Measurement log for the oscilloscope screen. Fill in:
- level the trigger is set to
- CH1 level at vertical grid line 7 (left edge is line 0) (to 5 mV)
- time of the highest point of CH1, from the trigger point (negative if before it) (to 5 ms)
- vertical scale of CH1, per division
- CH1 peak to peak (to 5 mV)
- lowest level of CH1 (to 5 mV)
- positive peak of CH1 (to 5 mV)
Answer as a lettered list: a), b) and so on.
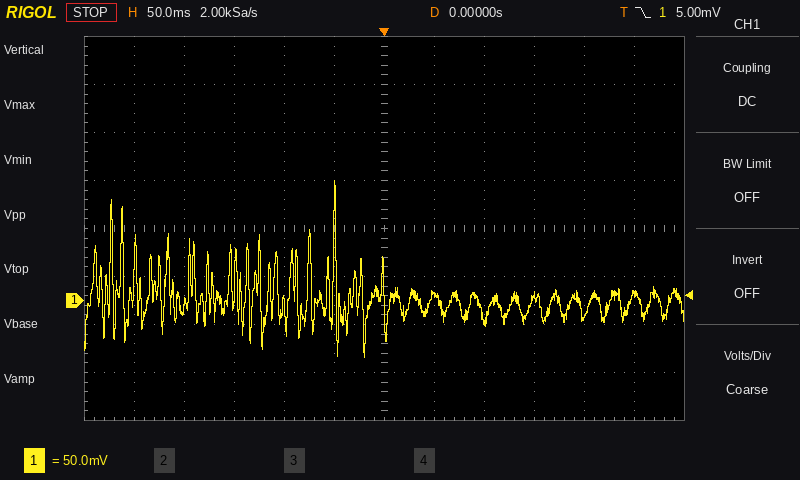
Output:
a) 5.00 mV
b) 5 mV
c) -50 ms
d) 50 mV
e) 185 mV
f) -60 mV
g) 125 mV
